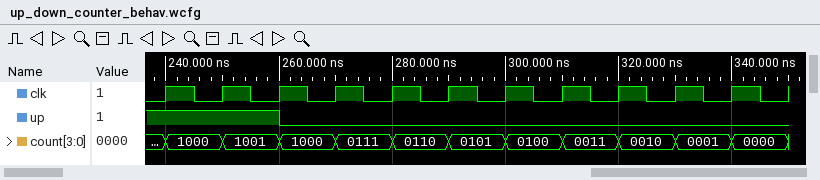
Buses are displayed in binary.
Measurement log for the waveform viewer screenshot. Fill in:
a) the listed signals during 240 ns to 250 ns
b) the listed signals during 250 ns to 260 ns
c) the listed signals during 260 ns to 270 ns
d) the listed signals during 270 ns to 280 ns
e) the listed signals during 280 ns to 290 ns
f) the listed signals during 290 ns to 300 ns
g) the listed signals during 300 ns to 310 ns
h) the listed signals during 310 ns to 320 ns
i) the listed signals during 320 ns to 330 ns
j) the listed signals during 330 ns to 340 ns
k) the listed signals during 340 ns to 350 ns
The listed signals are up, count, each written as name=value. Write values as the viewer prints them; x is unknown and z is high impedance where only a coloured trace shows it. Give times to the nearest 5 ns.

up=1, count=1000
up=1, count=1001
up=0, count=1000
up=0, count=0111
up=0, count=0110
up=0, count=0101
up=0, count=0100
up=0, count=0011
up=0, count=0010
up=0, count=0001
up=0, count=0000
